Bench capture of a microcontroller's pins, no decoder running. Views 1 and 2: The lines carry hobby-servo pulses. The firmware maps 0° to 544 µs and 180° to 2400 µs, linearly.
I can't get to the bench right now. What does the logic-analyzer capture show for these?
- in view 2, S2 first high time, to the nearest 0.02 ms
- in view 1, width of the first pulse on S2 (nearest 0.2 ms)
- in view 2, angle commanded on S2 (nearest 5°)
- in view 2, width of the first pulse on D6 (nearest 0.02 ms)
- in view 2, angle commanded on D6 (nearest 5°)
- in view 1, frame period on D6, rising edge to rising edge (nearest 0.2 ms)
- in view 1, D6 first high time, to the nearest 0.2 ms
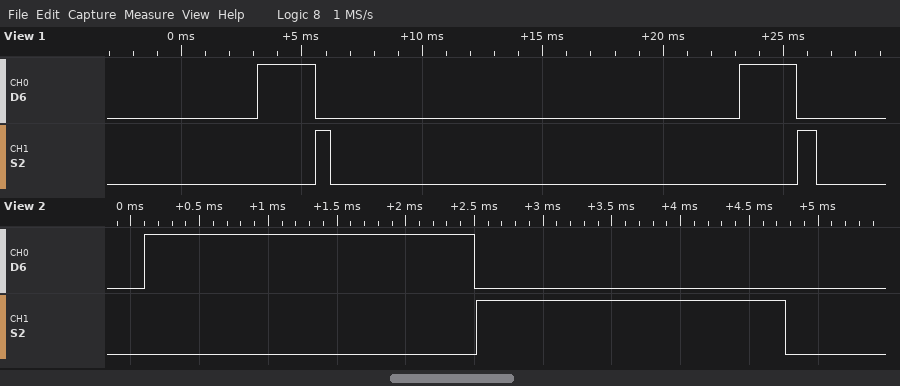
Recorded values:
2.26 ms
0.6 ms
165°
2.40 ms
180°
20.0 ms
2.4 ms
